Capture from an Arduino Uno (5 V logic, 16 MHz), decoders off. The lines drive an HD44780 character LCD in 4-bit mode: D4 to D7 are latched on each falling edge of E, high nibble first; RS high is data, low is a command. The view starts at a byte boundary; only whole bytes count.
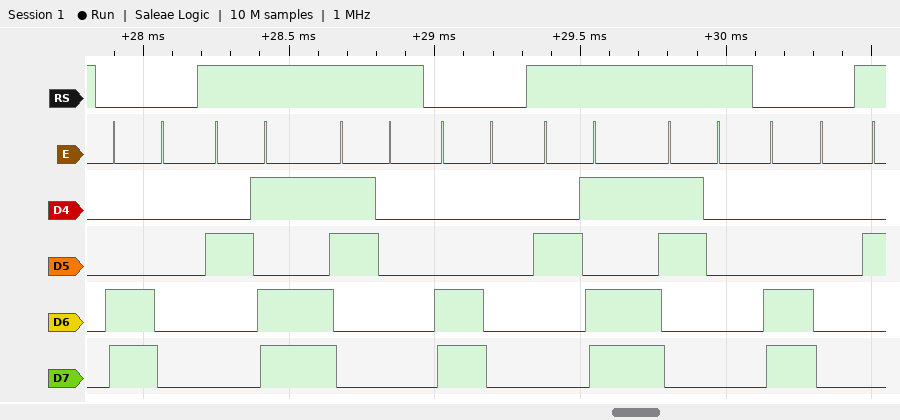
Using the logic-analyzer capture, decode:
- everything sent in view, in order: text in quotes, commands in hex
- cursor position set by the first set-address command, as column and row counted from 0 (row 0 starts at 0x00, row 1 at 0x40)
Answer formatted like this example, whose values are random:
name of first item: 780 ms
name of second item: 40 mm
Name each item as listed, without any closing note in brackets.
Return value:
everything sent in view, in order: text in quotes, commands in hex: 0xC0 "-0" 0xC0 "-0" 0xC0
cursor position set by the first set-address command, as column and row counted from 0: column 0, row 1
